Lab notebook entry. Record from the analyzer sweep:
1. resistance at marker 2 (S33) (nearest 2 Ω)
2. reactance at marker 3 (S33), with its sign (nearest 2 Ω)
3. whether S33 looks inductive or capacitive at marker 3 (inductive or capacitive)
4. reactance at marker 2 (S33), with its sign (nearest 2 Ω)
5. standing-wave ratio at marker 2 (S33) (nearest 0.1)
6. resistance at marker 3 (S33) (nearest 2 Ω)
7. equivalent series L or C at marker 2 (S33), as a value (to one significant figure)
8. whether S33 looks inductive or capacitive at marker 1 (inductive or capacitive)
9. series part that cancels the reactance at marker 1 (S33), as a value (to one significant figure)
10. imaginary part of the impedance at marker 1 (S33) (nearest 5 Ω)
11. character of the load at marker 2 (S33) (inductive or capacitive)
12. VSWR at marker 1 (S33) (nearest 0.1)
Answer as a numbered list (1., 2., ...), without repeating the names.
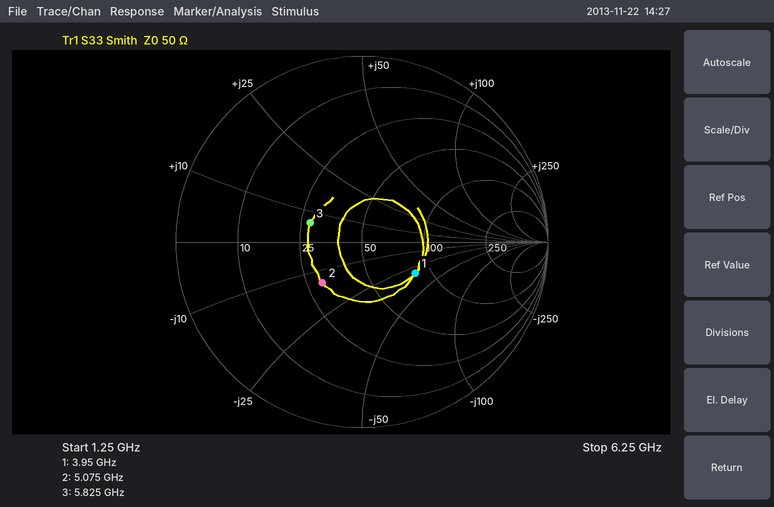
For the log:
1. 30 Ω
2. +6 Ω
3. inductive
4. -14 Ω
5. 1.9
6. 28 Ω
7. 2 pF
8. capacitive
9. 1 nH
10. -30 Ω
11. capacitive
12. 2.0
